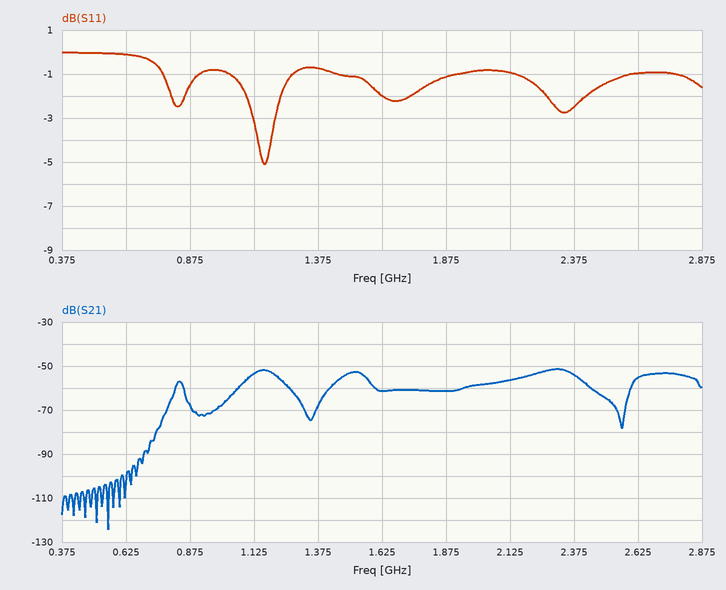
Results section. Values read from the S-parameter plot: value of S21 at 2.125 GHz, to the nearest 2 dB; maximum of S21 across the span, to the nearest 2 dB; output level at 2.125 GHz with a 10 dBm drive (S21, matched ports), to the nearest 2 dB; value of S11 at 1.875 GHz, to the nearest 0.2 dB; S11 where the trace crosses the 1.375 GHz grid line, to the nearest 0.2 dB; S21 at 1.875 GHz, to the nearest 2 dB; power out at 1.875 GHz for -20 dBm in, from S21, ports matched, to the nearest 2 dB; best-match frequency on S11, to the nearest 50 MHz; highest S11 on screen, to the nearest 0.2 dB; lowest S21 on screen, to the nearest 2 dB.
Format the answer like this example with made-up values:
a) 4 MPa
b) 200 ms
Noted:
a) -56 dB
b) -52 dB
c) -46 dBm
d) -1.2 dB
e) -0.8 dB
f) -62 dB
g) -82 dBm
h) 1.15 GHz
i) 0.0 dB
j) -124 dB
